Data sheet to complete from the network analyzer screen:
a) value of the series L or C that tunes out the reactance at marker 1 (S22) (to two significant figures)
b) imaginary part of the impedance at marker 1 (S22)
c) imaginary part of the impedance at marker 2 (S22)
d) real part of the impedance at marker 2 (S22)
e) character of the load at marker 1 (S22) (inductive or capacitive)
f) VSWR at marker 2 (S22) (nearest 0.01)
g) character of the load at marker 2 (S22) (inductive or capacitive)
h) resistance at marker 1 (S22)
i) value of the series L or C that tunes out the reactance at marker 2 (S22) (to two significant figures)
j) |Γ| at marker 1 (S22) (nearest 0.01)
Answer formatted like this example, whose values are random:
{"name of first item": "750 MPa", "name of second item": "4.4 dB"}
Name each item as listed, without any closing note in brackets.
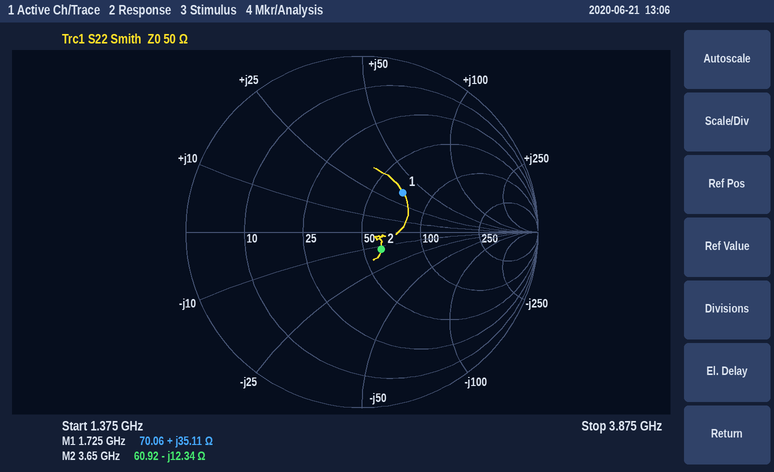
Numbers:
{"value of the series L or C that tunes out the reactance at marker 1 (S22)": "2.6 pF", "imaginary part of the impedance at marker 1": "+35.11 Ω", "imaginary part of the impedance at marker 2": "-12.34 Ω", "real part of the impedance at marker 2": "60.92 Ω", "character of the load at marker 1 (S22)": "inductive", "VSWR at marker 2 (S22)": "1.35", "character of the load at marker 2 (S22)": "capacitive", "resistance at marker 1": "70.06 Ω", "value of the series L or C that tunes out the reactance at marker 2 (S22)": "540 pH", "|Γ| at marker 1 (S22)": "0.32"}
